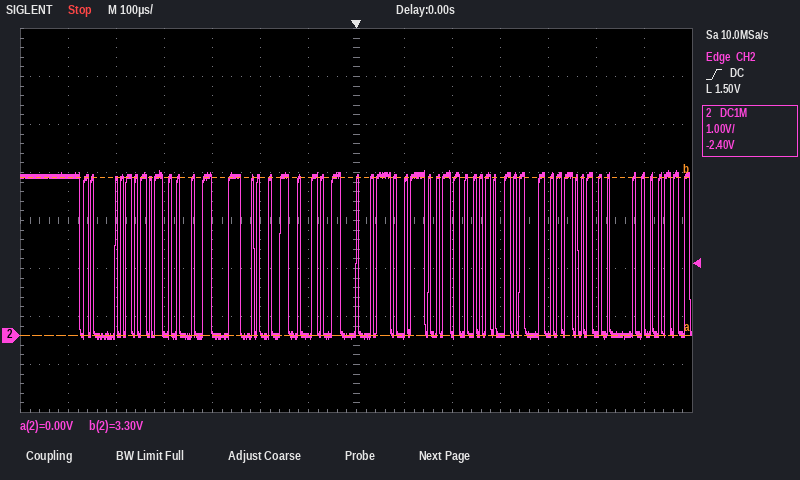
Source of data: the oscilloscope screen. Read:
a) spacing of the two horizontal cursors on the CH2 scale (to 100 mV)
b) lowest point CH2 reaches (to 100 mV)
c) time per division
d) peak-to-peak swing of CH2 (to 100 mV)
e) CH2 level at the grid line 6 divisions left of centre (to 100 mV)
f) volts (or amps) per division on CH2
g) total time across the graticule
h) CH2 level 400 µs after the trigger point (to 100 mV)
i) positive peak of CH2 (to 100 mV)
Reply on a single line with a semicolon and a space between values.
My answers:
3.3 V; -100 mV; 100 µs; 3.5 V; 3.3 V; 1 V; 1.4 ms; 0.0 V; 3.4 V
